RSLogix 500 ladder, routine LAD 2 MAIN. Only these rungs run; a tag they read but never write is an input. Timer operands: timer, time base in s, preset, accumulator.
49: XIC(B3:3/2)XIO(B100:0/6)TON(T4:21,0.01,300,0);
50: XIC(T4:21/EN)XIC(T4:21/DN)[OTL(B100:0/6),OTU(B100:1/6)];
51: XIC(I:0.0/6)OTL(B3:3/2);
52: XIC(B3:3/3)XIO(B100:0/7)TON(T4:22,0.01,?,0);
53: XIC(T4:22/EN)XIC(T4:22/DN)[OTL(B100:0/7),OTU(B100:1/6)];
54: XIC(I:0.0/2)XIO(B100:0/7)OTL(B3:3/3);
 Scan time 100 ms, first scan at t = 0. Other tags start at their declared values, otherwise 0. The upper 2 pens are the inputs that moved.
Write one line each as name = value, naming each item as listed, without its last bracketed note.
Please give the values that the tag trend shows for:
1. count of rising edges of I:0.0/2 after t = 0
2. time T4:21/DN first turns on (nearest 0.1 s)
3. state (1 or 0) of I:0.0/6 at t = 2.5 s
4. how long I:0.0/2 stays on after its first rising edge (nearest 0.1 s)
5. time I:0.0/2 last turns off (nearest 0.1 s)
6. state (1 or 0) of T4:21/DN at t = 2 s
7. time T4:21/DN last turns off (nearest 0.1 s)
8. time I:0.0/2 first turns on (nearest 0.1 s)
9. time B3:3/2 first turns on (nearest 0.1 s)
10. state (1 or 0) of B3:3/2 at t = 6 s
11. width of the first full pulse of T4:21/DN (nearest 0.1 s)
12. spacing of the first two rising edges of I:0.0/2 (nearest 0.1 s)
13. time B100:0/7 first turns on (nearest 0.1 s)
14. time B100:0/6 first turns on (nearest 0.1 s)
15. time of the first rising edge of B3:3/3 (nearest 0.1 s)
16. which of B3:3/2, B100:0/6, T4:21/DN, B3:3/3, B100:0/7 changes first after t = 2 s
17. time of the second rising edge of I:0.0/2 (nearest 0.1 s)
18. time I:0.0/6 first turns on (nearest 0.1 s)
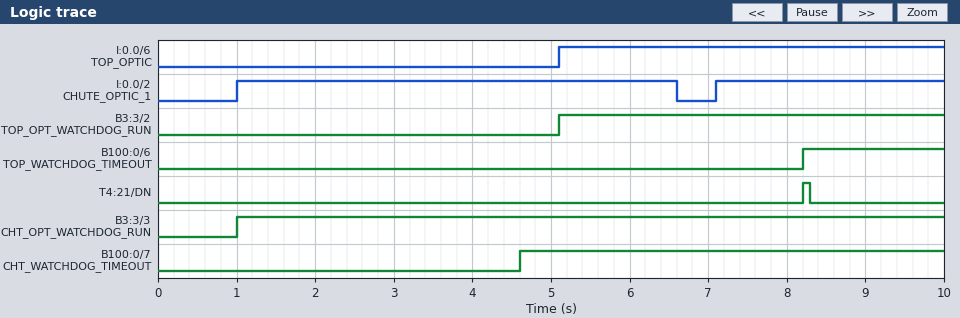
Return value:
count of rising edges of I:0.0/2 after t = 0 = 2
time T4:21/DN first turns on = 8.2 s
state (1 or 0) of I:0.0/6 at t = 2.5 s = 0
how long I:0.0/2 stays on after its first rising edge = 5.6 s
time I:0.0/2 last turns off = 6.6 s
state (1 or 0) of T4:21/DN at t = 2 s = 0
time T4:21/DN last turns off = 8.3 s
time I:0.0/2 first turns on = 1.0 s
time B3:3/2 first turns on = 5.1 s
state (1 or 0) of B3:3/2 at t = 6 s = 1
width of the first full pulse of T4:21/DN = 0.1 s
spacing of the first two rising edges of I:0.0/2 = 6.1 s
time B100:0/7 first turns on = 4.6 s
time B100:0/6 first turns on = 8.2 s
time of the first rising edge of B3:3/3 = 1.0 s
which of B3:3/2, B100:0/6, T4:21/DN, B3:3/3, B100:0/7 changes first after t = 2 s = B100:0/7
time of the second rising edge of I:0.0/2 = 7.1 s
time I:0.0/6 first turns on = 5.1 s
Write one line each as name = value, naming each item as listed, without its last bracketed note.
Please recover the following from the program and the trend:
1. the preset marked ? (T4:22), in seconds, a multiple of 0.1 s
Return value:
the preset marked ? (T4:22), in seconds, a multiple of 0.1 s = 3.5 s
